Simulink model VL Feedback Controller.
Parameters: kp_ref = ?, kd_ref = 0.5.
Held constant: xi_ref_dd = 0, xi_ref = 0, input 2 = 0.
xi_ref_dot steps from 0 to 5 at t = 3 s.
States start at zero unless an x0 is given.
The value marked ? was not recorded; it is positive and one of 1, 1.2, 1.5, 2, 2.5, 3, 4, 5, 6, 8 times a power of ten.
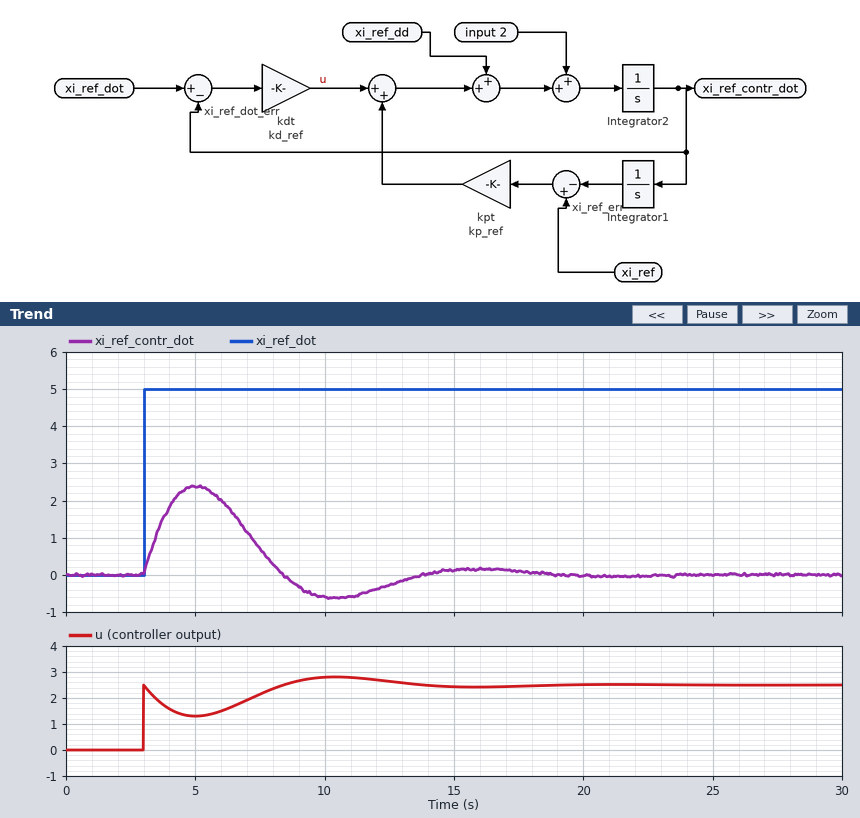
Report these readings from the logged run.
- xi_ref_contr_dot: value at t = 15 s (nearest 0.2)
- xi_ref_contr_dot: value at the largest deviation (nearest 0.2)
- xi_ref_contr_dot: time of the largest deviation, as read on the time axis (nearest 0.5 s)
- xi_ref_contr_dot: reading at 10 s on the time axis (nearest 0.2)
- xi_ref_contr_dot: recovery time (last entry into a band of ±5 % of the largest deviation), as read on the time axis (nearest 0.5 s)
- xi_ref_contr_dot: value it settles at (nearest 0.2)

0.2
2.4
5.0 s
-0.6
17.0 s
0.0
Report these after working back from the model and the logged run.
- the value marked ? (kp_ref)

0.4
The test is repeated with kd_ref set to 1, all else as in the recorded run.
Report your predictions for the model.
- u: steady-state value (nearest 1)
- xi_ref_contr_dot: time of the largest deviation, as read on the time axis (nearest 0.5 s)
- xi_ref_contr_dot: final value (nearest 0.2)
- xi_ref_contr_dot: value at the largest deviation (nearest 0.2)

5
4.5 s
0.0
3.4
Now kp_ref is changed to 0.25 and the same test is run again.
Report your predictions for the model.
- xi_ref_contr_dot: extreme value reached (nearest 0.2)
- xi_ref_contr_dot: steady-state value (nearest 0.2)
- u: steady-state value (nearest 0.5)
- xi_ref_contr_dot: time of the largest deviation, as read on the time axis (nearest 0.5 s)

2.8
0.0
2.5
5.5 s
